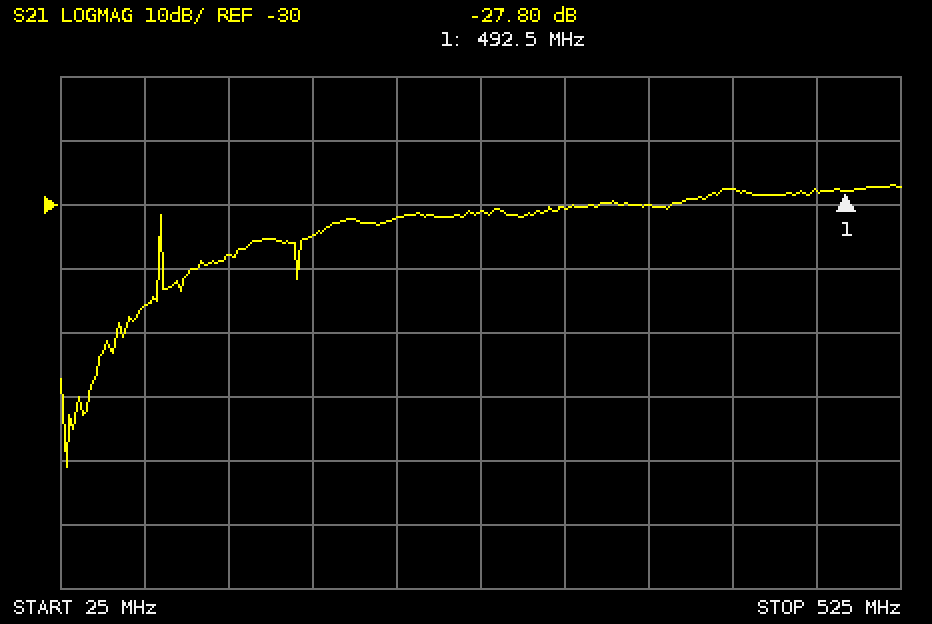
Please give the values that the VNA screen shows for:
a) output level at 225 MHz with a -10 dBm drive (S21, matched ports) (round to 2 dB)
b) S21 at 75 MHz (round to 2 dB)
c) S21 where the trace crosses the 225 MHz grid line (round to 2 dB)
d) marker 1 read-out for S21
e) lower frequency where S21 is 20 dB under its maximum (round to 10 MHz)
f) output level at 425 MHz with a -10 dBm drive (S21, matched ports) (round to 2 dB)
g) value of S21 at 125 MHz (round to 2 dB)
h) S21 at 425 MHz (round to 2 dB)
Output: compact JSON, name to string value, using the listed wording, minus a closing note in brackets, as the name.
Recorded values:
{"output level at 225 MHz with a -10 dBm drive (S21, matched ports)": "-42 dBm", "S21 at 75 MHz": "-46 dB", "S21 where the trace crosses the 225 MHz grid line": "-32 dB", "marker 1 read-out for S21": "-27.80 dB", "lower frequency where S21 is 20 dB under its maximum": "70 MHz", "output level at 425 MHz with a -10 dBm drive (S21, matched ports)": "-38 dBm", "value of S21 at 125 MHz": "-38 dB", "S21 at 425 MHz": "-28 dB"}
